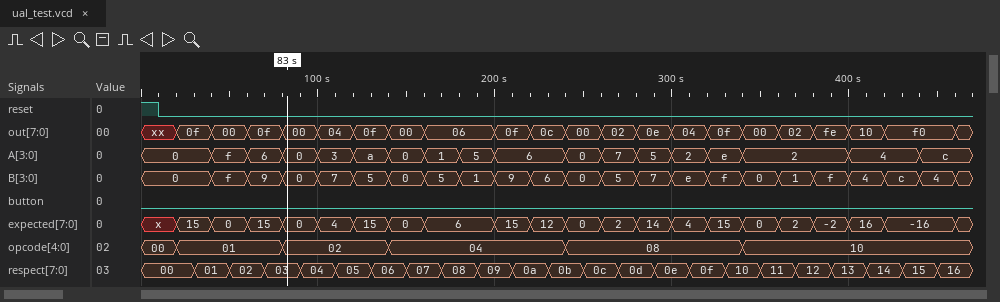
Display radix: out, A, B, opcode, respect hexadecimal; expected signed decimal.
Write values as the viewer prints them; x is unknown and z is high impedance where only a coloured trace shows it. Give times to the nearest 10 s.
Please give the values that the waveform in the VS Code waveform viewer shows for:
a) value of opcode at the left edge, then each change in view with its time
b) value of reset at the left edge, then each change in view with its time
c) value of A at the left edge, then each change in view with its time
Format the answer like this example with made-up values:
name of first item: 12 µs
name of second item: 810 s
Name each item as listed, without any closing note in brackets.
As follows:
value of opcode at the left edge, then each change in view with its time: 00, 01 at 20 s, 02 at 80 s, 04 at 140 s, 08 at 240 s, 10 at 340 s
value of reset at the left edge, then each change in view with its time: 1, 0 at 10 s
value of A at the left edge, then each change in view with its time: 0, f at 40 s, 6 at 60 s, 0 at 80 s, 3 at 100 s, a at 120 s, 0 at 140 s, 1 at 160 s, 5 at 180 s, 6 at 200 s, 0 at 240 s, 7 at 260 s, 5 at 280 s, 2 at 300 s, e at 320 s, 2 at 340 s, 4 at 400 s, c at 440 s
